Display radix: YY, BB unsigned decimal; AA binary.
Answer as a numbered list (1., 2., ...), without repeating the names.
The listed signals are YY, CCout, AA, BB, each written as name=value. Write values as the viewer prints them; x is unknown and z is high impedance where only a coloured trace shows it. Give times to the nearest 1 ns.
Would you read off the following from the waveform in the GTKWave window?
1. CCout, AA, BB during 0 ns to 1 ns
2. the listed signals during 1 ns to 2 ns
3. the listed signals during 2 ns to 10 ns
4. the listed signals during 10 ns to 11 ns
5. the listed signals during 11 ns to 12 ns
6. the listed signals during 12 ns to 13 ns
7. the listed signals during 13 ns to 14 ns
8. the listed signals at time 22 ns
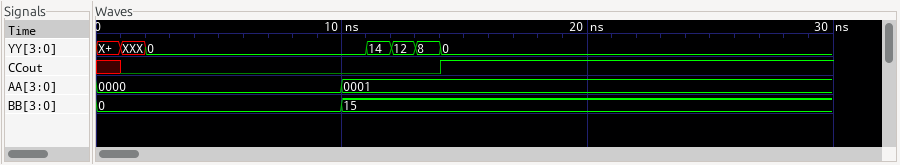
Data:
1. CCout=x, AA=0000, BB=0
2. YY=XXX, CCout=0, AA=0000, BB=0
3. YY=0, CCout=0, AA=0000, BB=0
4. YY=0, CCout=0, AA=0001, BB=15
5. YY=14, CCout=0, AA=0001, BB=15
6. YY=12, CCout=0, AA=0001, BB=15
7. YY=8, CCout=0, AA=0001, BB=15
8. YY=0, CCout=1, AA=0001, BB=15
